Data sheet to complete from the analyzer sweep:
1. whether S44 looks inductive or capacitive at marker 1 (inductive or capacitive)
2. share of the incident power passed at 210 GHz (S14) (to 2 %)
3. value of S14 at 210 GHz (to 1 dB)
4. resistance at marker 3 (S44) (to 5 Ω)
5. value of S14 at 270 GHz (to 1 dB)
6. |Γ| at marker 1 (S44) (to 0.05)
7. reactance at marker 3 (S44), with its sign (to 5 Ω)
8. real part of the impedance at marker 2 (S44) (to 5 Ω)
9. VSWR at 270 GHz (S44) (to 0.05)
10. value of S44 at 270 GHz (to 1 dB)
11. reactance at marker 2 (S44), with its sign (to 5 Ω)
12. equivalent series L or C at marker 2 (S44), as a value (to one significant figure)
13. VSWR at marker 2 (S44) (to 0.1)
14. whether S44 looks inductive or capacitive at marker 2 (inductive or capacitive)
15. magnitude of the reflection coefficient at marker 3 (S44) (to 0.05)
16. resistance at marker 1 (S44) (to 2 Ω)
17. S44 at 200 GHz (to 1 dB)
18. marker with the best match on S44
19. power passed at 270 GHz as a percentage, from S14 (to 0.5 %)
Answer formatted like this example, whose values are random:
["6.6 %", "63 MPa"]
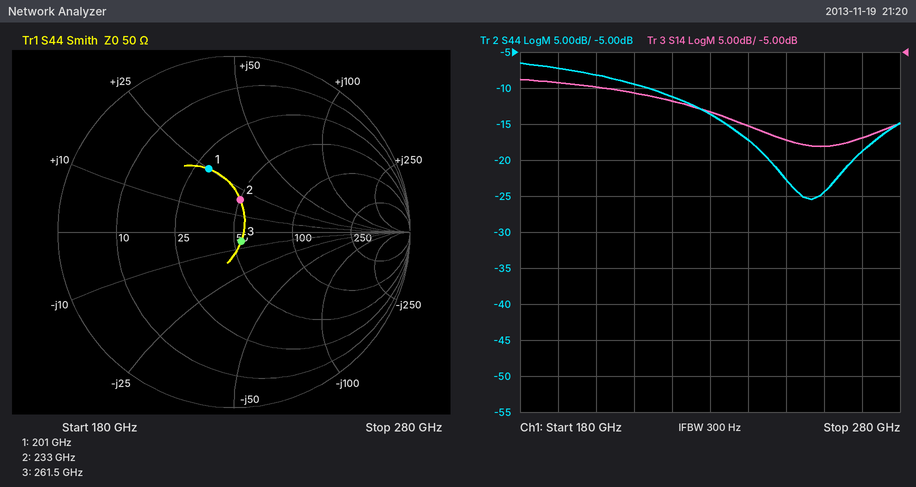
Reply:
["inductive", "8 %", "-11 dB", "55 Ω", "-17 dB", "0.40", "-5 Ω", "50 Ω", "1.25", "-19 dB", "+20 Ω", "10 pH", "1.5", "inductive", "0.05", "30 Ω", "-8 dB", "marker 3", "2.0 %"]
